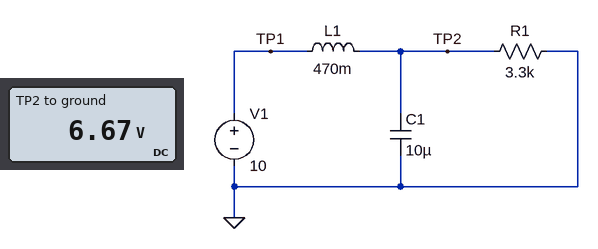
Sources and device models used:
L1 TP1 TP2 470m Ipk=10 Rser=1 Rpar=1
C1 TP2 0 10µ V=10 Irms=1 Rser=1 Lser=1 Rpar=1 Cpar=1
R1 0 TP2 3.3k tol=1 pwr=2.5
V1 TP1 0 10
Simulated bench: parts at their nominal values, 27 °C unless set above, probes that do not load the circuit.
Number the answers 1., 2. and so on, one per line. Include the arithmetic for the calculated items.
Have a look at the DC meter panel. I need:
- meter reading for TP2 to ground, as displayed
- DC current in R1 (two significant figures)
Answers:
1. 6.67 V
2. (6.67 V) / 3.3 kΩ = 2.0 mA
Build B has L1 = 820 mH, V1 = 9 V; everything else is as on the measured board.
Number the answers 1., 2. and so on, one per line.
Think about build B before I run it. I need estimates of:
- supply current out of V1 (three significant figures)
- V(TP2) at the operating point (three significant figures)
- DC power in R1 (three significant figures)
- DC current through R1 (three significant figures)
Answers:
1. 6.00 A
2. 6.00 V
3. 10.9 mW
4. 1.82 mA
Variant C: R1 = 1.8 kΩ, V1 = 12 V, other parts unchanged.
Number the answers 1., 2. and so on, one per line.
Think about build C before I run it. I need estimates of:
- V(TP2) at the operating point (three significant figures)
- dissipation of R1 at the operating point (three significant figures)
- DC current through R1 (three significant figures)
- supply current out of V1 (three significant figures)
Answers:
1. 8.00 V
2. 35.5 mW
3. 4.44 mA
4. 8.00 A
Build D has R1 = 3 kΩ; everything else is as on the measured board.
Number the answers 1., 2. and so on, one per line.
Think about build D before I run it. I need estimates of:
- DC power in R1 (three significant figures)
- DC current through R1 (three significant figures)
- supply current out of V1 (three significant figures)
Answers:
1. 14.8 mW
2. 2.22 mA
3. 6.67 A
